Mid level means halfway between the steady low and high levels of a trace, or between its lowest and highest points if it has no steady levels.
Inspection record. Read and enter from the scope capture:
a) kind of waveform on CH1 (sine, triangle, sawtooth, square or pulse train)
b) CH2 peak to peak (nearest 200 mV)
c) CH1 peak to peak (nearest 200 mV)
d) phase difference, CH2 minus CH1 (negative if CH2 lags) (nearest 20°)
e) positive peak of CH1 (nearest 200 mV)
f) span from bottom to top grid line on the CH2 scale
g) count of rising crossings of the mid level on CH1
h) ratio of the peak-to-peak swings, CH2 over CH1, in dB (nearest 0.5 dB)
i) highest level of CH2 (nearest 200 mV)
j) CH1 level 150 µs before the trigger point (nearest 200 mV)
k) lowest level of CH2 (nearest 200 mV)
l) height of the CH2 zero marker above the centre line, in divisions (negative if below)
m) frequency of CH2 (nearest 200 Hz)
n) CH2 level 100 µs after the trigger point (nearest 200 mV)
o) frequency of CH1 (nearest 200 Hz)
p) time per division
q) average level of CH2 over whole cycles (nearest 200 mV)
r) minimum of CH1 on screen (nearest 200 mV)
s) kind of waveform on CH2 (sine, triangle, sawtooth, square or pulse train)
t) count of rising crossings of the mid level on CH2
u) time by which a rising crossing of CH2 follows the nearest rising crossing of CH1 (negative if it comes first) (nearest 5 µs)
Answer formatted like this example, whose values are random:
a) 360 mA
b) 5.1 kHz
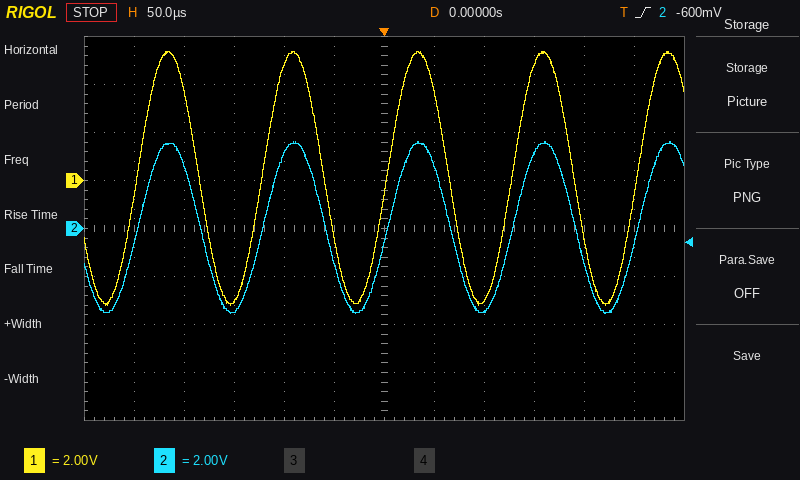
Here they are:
a) sine
b) 7.2 V
c) 10.6 V
d) 0°
e) 5.4 V
f) 16 V
g) 5
h) -3.5 dB
i) 3.6 V
j) -5.0 V
k) -3.6 V
l) 0.0 div
m) 8.0 kHz
n) -3.4 V
o) 8.0 kHz
p) 50 µs
q) 0.0 V
r) -5.2 V
s) sine
t) 5
u) 0 µs
